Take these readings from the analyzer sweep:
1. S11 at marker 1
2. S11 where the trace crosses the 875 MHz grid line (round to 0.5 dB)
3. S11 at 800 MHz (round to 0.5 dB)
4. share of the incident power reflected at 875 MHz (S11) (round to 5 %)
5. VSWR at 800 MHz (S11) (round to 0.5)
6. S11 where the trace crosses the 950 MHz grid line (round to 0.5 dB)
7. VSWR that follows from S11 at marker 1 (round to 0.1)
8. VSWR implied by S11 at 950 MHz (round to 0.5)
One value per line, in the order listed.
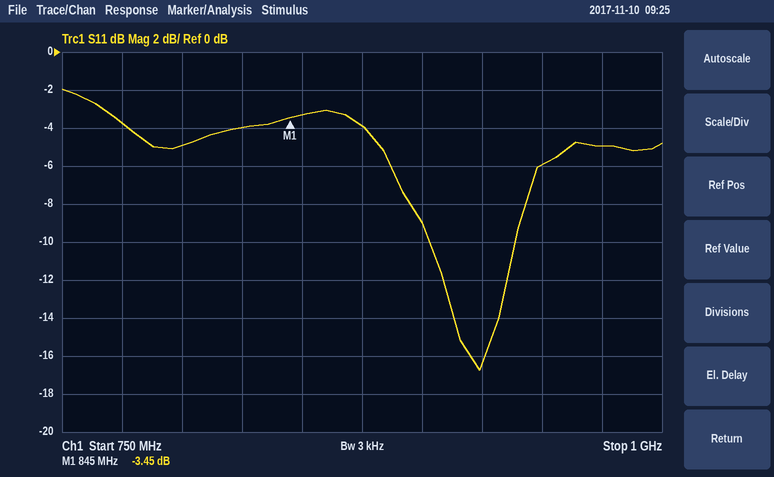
-3.45 dB
-4.0 dB
-5.0 dB
40 %
3.5
-6.0 dB
5.1
3.0
